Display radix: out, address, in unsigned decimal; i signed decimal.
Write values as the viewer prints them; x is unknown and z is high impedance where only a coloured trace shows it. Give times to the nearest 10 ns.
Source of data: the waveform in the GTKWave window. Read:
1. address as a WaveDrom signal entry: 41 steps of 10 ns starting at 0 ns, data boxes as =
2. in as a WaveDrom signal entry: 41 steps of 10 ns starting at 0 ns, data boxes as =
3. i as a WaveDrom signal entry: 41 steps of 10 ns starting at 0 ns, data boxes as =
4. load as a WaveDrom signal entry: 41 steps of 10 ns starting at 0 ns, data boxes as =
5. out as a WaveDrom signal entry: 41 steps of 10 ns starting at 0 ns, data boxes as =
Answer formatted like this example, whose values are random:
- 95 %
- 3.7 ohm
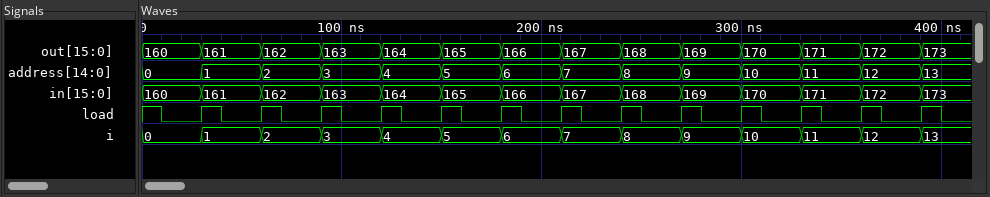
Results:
- {name: 'address', wave: '=..=..=..=..=..=..=..=..=..=..=..=..=..=.', data: '0 1 2 3 4 5 6 7 8 9 10 11 12 13'}
- {name: 'in', wave: '=..=..=..=..=..=..=..=..=..=..=..=..=..=.', data: '160 161 162 163 164 165 166 167 168 169 170 171 172 173'}
- {name: 'i', wave: '=..=..=..=..=..=..=..=..=..=..=..=..=..=.', data: '0 1 2 3 4 5 6 7 8 9 10 11 12 13'}
- {name: 'load', wave: '10.10.10.10.10.10.10.10.10.10.10.10.10.10'}
- {name: 'out', wave: '=..=..=..=..=..=..=..=..=..=..=..=..=..=.', data: '160 161 162 163 164 165 166 167 168 169 170 171 172 173'}
